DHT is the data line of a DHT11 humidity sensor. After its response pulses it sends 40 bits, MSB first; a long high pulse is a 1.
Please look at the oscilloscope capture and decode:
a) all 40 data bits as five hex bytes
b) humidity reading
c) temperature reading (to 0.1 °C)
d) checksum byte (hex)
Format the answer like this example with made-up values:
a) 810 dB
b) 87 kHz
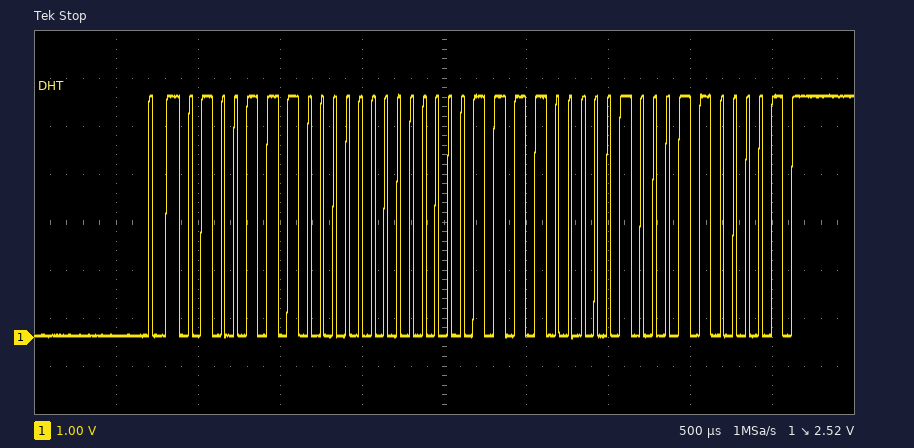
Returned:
a) 4E 00 0F 04 61
b) 78 %
c) 15.4 °C
d) 0x61
